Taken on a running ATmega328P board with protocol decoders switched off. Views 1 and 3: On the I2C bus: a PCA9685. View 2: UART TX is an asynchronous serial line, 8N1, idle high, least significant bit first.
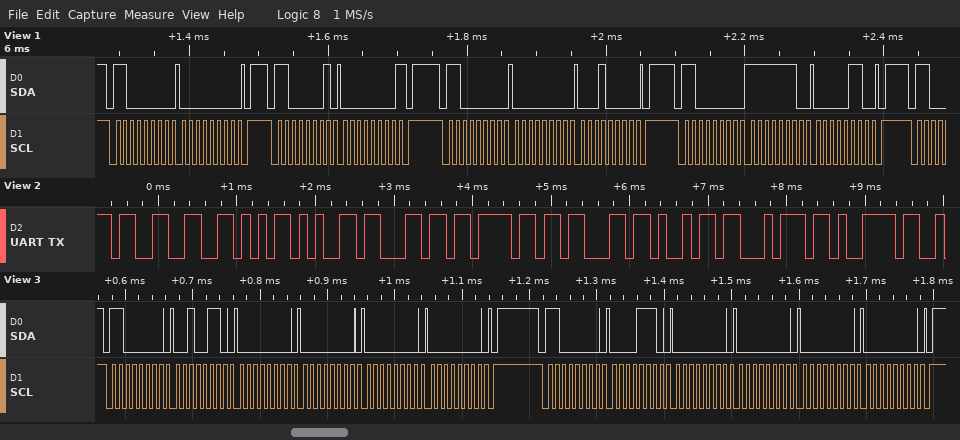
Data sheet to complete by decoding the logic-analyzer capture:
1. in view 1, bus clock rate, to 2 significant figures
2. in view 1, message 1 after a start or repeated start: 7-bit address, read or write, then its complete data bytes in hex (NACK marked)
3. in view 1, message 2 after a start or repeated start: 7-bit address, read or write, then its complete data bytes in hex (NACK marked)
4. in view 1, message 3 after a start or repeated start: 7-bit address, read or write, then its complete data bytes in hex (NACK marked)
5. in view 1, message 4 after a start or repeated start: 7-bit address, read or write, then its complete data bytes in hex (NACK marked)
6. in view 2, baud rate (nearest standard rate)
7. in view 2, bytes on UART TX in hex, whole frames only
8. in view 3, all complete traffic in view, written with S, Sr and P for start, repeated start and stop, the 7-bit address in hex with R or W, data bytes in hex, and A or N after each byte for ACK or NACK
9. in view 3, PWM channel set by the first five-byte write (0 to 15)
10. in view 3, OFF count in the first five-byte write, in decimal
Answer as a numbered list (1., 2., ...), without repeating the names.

1. 100 kHz
2. 0x60 write: 00
3. 0x60 read: 00 NACK
4. 0x60 write: 00 10
5. 0x60 write: FE 06
6. 9600 baud
7. 33 56 65 6C 6F 63 69 74 79
8. S 60W A 26 A 00 A 00 A 00 A 00 A P S 60W A 0E A 00 A 00 A 00 A 00 A P
9. 8
10. 0
